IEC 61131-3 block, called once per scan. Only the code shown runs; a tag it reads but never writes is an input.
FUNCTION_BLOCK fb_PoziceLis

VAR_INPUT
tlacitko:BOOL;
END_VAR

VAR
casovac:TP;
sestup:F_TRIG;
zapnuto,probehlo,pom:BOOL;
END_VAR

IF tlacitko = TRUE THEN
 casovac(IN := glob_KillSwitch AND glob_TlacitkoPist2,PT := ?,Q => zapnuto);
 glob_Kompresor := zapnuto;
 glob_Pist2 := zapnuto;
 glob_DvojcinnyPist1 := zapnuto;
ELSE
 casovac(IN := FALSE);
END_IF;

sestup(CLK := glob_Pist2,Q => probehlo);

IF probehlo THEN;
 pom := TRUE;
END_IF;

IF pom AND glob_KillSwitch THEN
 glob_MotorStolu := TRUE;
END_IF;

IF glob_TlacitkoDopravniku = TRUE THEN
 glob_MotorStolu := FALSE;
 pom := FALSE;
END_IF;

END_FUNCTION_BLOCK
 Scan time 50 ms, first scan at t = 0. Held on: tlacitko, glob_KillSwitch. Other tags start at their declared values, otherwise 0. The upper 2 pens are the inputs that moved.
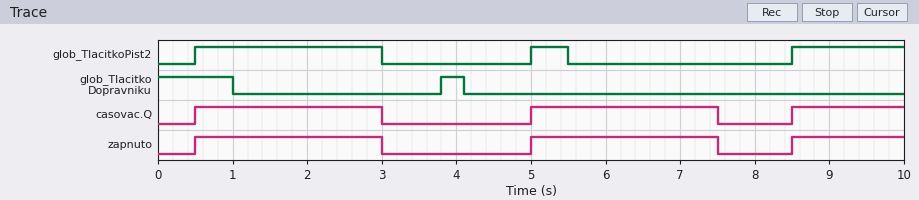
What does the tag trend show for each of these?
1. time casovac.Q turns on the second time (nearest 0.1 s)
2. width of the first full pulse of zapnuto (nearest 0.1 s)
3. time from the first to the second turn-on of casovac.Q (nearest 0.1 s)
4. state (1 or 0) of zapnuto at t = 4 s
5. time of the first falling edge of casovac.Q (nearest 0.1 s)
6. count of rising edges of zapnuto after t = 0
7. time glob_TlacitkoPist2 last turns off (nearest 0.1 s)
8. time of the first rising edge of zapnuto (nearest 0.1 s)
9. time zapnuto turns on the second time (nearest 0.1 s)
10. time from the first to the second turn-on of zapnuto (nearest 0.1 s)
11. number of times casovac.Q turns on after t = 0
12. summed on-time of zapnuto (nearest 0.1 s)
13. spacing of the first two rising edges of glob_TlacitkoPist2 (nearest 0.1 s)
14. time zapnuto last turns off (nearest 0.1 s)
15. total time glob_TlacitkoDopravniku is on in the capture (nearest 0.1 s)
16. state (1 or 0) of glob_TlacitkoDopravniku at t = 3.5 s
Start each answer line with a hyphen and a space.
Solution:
- 5.0 s
- 2.5 s
- 4.5 s
- 0
- 3.0 s
- 3
- 5.5 s
- 0.5 s
- 5.0 s
- 4.5 s
- 3
- 6.5 s
- 4.5 s
- 7.5 s
- 1.3 s
- 0
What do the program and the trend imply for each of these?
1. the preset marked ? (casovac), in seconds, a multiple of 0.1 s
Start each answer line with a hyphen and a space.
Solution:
- 2.5 s
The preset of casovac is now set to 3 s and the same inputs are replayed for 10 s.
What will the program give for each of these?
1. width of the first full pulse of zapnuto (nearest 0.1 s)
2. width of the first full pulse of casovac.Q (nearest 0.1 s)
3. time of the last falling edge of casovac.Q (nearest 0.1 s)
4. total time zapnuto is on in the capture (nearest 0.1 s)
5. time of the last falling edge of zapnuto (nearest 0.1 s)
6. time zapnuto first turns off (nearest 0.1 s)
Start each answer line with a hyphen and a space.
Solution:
- 3.0 s
- 3.0 s
- 8.0 s
- 7.5 s
- 8.0 s
- 3.5 s
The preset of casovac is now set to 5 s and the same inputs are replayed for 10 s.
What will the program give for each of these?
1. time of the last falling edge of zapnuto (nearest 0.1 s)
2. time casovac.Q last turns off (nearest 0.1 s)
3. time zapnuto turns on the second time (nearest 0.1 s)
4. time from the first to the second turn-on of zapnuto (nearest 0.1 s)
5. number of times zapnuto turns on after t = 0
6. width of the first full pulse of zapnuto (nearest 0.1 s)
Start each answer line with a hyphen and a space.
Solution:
- 5.5 s
- 5.5 s
- 8.5 s
- 8.0 s
- 2
- 5.0 s
